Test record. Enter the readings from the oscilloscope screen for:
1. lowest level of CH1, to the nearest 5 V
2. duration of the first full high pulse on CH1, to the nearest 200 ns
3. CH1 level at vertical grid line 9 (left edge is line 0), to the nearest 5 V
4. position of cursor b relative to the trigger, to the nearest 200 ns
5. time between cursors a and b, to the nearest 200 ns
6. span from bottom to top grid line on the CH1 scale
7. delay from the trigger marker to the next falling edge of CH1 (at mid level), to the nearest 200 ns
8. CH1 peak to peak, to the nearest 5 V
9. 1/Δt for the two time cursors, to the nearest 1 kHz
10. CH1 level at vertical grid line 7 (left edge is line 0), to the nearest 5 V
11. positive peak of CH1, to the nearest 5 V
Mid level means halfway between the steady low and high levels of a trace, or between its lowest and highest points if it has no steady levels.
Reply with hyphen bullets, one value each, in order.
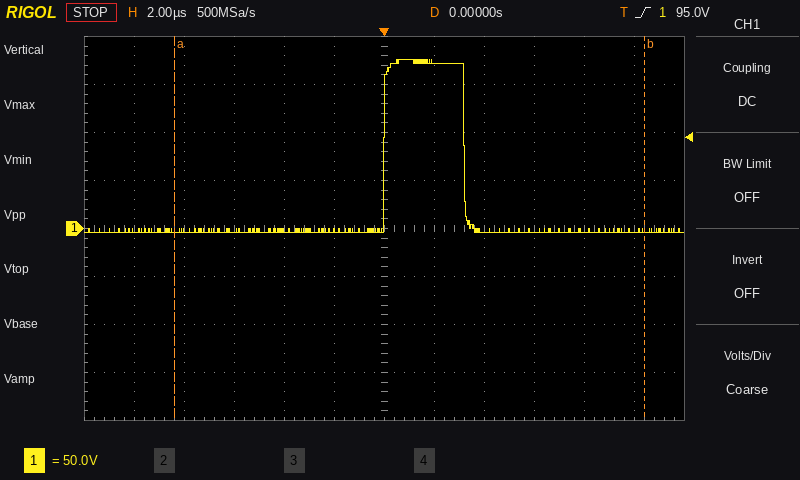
- -5 V
- 3.2 µs
- -5 V
- +10.4 µs
- 18.8 µs
- 400 V
- 3.2 µs
- 180 V
- 53 kHz
- 175 V
- 175 V
